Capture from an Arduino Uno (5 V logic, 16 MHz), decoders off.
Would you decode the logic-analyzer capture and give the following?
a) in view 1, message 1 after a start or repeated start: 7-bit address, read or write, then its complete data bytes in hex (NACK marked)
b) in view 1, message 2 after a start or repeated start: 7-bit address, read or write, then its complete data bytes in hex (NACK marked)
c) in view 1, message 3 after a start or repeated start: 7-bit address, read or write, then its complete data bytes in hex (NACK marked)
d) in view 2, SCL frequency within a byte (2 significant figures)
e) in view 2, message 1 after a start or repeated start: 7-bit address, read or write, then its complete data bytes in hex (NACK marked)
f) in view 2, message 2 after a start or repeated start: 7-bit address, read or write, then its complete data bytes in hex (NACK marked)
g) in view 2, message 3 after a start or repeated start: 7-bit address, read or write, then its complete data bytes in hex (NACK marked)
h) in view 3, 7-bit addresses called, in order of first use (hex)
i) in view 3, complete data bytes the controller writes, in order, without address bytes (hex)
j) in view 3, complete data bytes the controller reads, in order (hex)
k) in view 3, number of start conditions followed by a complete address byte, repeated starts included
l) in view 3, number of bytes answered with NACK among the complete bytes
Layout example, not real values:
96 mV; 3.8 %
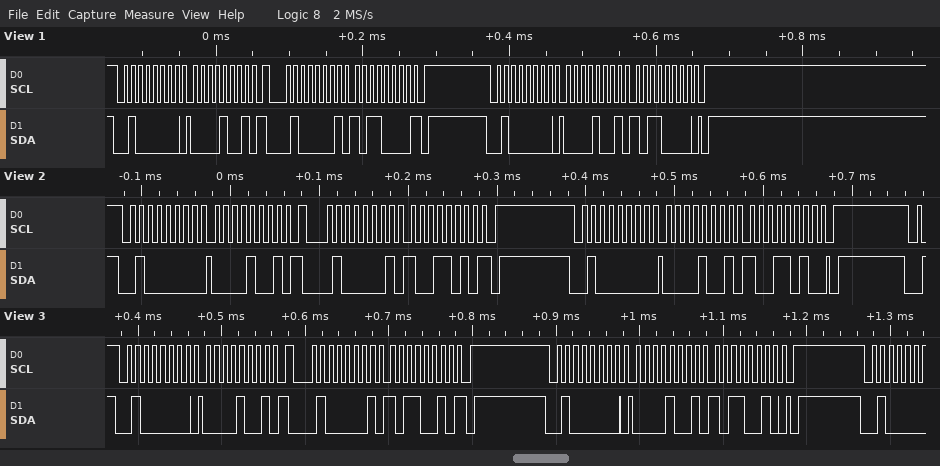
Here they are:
0x20 write: 09; 0x20 read: B0 NACK; 0x20 write: 09 B0; 100 kHz; 0x20 write: 09; 0x20 read: 9A NACK; 0x20 write: 09 9A; 0x20; 09 09 B2; B2; 3; 1
